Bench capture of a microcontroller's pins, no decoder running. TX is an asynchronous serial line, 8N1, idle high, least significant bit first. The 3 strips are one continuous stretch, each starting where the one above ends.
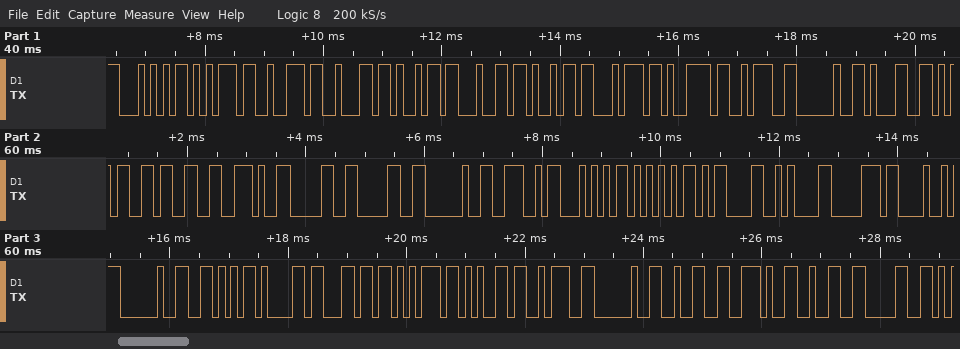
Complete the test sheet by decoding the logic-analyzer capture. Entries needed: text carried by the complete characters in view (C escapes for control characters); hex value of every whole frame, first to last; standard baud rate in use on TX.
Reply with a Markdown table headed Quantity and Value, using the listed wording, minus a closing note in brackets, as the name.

| Quantity | Value |
|---|---|
| text carried by the complete characters in view | "Turbidity: 153.00 NTU\r\npH Value: 2.20" |
| hex value of every whole frame, first to last | 54 75 72 62 69 64 69 74 79 3A 20 31 35 33 2E 30 30 20 4E 54 55 0D 0A 70 48 20 56 61 6C 75 65 3A 20 32 2E 32 30 |
| standard baud rate in use on TX | 9600 baud |
